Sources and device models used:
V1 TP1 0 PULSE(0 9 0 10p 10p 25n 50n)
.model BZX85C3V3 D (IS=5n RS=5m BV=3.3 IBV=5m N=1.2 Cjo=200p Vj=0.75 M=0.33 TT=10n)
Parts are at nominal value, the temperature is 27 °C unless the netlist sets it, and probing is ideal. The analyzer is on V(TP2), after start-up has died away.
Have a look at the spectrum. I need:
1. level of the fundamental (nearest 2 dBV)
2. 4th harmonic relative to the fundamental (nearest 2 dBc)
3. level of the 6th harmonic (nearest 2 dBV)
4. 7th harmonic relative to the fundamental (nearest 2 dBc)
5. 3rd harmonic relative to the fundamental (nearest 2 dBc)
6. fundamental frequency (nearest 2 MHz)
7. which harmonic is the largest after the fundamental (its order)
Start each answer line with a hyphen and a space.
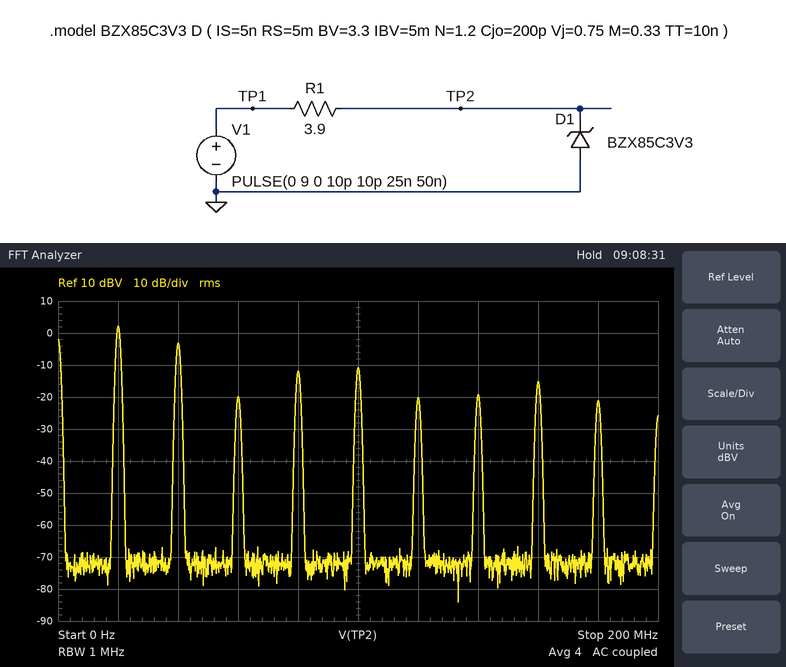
- 2 dBV
- -14 dBc
- -20 dBV
- -22 dBc
- -22 dBc
- 20 MHz
- 2
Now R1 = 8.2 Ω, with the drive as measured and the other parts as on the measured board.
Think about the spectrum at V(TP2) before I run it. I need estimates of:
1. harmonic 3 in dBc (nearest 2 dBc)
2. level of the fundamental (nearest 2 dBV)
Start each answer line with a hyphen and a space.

- -20 dBc
- 2 dBV
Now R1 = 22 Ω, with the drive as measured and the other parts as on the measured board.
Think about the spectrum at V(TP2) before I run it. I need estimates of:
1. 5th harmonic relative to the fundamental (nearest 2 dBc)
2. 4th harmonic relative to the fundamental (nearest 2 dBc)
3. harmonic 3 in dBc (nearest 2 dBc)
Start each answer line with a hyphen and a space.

- -14 dBc
- -16 dBc
- -16 dBc
